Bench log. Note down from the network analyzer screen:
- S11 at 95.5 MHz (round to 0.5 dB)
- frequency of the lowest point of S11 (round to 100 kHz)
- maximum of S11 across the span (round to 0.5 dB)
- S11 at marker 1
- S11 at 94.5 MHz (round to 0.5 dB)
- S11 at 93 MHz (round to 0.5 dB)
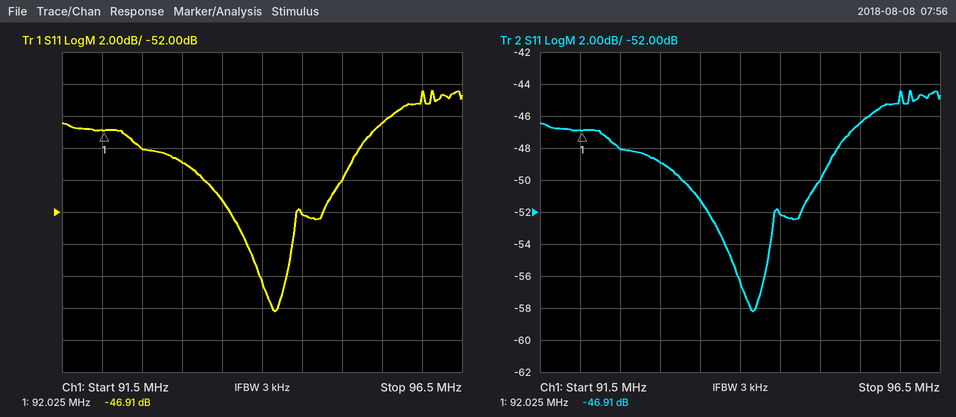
-46.5 dB
94.2 MHz
-44.5 dB
-46.91 dB
-52.0 dB
-49.0 dB
